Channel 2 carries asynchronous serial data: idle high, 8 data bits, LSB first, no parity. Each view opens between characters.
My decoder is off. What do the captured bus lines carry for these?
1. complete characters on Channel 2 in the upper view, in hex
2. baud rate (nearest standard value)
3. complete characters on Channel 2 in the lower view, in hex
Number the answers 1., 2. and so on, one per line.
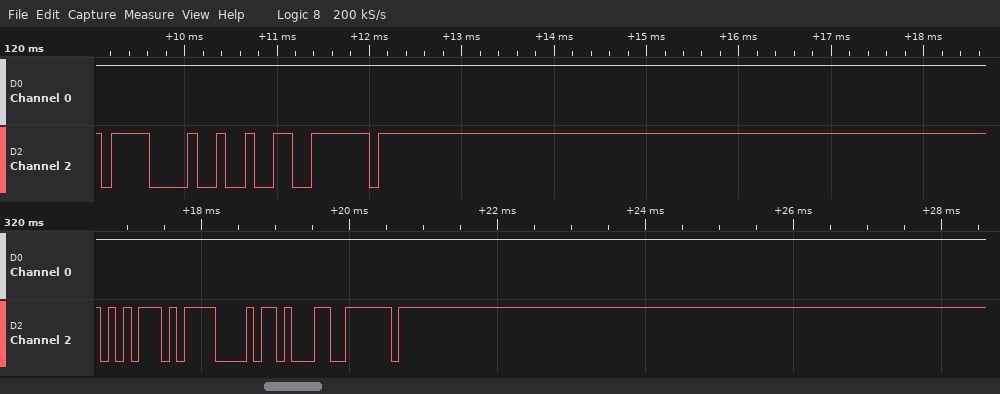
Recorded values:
1. 0F, 92, 7E
2. 9600 baud
3. 75, 0F, 8B, 7E
